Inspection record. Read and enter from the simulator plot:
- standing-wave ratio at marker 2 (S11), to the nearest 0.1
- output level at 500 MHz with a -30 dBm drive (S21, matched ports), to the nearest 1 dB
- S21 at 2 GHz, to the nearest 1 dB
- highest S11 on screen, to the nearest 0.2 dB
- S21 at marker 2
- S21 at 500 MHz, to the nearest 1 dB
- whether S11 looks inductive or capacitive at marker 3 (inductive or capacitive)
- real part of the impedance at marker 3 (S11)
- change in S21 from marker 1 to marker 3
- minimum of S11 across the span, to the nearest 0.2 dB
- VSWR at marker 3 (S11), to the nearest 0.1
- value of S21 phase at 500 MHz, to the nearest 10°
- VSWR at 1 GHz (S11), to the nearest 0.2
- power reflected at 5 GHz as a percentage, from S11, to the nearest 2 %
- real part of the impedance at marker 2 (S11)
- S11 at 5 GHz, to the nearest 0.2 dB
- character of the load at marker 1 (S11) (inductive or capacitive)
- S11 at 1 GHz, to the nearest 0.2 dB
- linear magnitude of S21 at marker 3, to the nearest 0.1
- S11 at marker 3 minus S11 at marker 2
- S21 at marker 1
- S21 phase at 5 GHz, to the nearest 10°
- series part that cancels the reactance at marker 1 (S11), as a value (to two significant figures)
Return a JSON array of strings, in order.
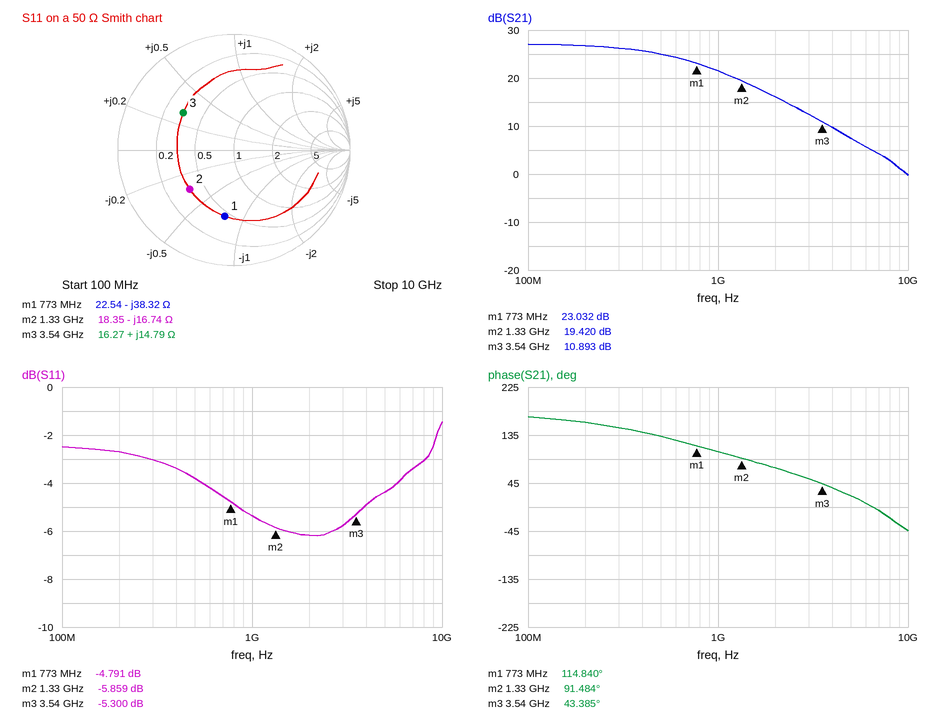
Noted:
["3.1", "-5 dBm", "16 dB", "-1.4 dB", "19.420 dB", "25 dB", "inductive", "16.27 Ω", "-12.139 dB", "-6.2 dB", "3.4", "130°", "3.4", "36 %", "18.35 Ω", "-4.4 dB", "capacitive", "-5.4 dB", "3.5", "0.559 dB", "23.032 dB", "20°", "7.9 nH"]
